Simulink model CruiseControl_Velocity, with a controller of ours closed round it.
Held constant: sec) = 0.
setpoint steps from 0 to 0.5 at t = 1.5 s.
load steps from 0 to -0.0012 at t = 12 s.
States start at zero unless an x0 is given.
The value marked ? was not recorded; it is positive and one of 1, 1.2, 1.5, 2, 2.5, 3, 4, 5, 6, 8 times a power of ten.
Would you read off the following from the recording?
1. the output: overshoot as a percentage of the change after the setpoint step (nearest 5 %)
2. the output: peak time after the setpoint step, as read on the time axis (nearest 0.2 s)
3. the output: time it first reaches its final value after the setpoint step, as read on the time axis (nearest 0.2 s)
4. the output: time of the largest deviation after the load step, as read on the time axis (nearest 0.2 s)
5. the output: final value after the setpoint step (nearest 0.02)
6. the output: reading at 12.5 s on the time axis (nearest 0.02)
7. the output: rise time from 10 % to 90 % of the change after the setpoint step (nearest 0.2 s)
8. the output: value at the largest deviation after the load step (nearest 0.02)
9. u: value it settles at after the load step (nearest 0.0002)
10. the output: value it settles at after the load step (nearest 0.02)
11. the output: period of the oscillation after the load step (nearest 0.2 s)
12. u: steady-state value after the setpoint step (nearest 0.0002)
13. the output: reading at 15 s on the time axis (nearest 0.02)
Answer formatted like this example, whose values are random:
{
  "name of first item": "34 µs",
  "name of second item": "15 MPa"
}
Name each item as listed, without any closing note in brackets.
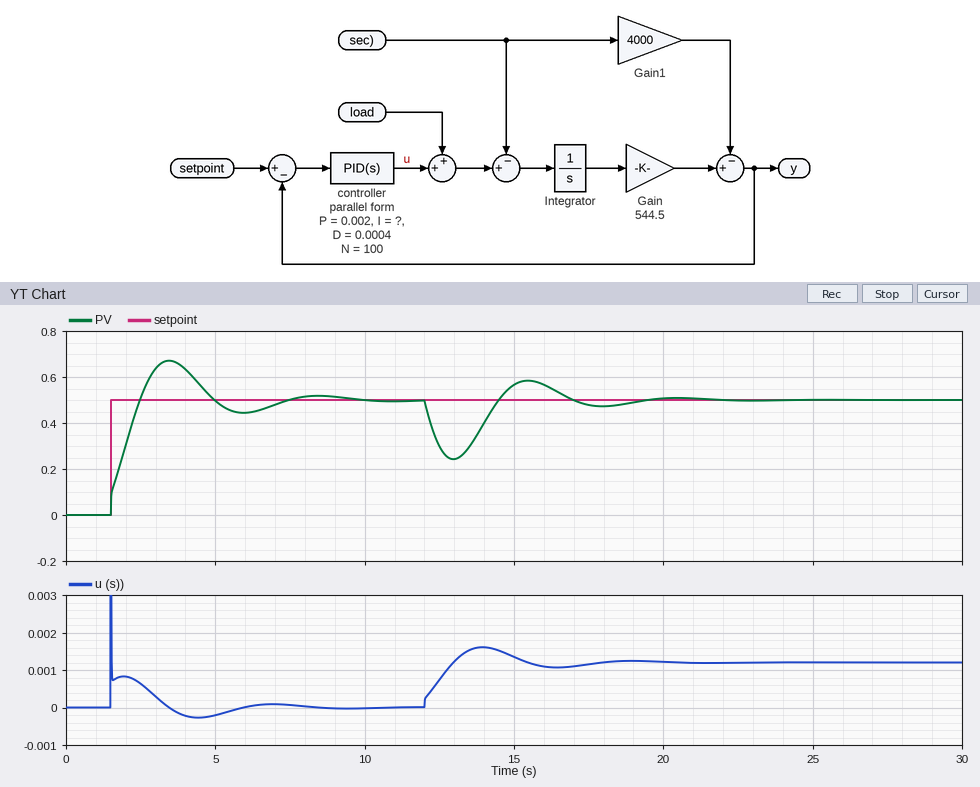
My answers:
{
  "the output: overshoot as a percentage of the change after the setpoint step": "35 %",
  "the output: peak time after the setpoint step, as read on the time axis": "3.4 s",
  "the output: time it first reaches its final value after the setpoint step, as read on the time axis": "2.4 s",
  "the output: time of the largest deviation after the load step, as read on the time axis": "13.0 s",
  "the output: final value after the setpoint step": "0.50",
  "the output: reading at 12.5 s on the time axis": "0.30",
  "the output: rise time from 10 % to 90 % of the change after the setpoint step": "0.8 s",
  "the output: value at the largest deviation after the load step": "0.24",
  "u: value it settles at after the load step": "0.0012",
  "the output: value it settles at after the load step": "0.50",
  "the output: period of the oscillation after the load step": "5.0 s",
  "u: steady-state value after the setpoint step": "0.0000",
  "the output: reading at 15 s on the time axis": "0.56"
}
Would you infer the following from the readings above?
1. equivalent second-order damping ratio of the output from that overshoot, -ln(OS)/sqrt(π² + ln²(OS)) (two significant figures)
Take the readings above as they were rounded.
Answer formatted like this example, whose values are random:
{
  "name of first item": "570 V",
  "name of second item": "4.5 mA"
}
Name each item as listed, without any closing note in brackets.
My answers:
{
  "equivalent second-order damping ratio of the output from that overshoot, -ln(OS)/sqrt(π² + ln²(OS))": "0.32"
}
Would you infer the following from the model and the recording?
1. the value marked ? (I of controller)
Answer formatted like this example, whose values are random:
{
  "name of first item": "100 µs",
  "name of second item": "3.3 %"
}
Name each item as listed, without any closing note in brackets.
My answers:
{
  "the value marked ?": "0.004"
}
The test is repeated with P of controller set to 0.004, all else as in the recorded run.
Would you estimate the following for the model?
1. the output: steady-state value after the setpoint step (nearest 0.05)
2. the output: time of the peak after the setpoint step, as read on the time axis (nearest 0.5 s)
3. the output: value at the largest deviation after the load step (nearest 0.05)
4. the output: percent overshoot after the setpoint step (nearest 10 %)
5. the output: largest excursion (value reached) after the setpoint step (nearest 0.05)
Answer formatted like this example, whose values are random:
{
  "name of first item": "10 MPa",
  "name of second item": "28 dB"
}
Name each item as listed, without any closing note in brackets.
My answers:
{
  "the output: steady-state value after the setpoint step": "0.50",
  "the output: time of the peak after the setpoint step, as read on the time axis": "3.0 s",
  "the output: value at the largest deviation after the load step": "0.30",
  "the output: percent overshoot after the setpoint step": "20 %",
  "the output: largest excursion (value reached) after the setpoint step": "0.60"
}
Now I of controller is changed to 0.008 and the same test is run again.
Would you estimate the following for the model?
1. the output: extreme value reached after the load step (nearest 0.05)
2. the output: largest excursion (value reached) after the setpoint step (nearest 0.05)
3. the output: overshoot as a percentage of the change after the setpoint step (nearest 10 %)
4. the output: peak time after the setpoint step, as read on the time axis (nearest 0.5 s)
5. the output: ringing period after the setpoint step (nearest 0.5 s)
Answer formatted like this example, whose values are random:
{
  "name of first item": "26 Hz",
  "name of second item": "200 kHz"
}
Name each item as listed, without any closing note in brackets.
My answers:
{
  "the output: extreme value reached after the load step": "0.30",
  "the output: largest excursion (value reached) after the setpoint step": "0.70",
  "the output: overshoot as a percentage of the change after the setpoint step": "40 %",
  "the output: peak time after the setpoint step, as read on the time axis": "3.0 s",
  "the output: ringing period after the setpoint step": "3.5 s"
}
